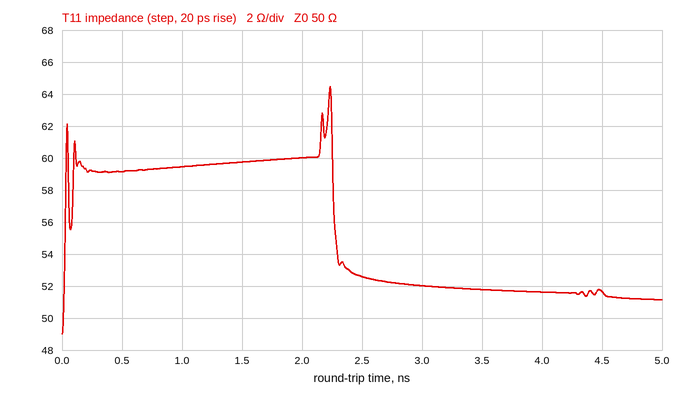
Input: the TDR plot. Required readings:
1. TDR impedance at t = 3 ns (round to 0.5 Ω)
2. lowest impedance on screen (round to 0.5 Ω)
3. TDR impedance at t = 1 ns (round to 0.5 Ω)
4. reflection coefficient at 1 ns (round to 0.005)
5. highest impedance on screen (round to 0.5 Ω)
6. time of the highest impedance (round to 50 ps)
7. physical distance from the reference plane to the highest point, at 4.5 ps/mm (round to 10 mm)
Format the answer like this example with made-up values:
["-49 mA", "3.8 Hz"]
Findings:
["52.0 Ω", "49.0 Ω", "59.5 Ω", "+0.085", "64.5 Ω", "2.25 ns", "250 mm"]
